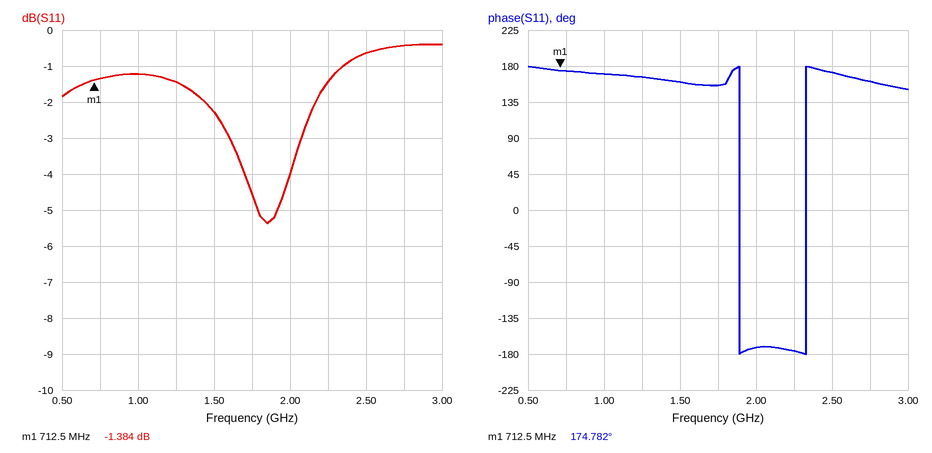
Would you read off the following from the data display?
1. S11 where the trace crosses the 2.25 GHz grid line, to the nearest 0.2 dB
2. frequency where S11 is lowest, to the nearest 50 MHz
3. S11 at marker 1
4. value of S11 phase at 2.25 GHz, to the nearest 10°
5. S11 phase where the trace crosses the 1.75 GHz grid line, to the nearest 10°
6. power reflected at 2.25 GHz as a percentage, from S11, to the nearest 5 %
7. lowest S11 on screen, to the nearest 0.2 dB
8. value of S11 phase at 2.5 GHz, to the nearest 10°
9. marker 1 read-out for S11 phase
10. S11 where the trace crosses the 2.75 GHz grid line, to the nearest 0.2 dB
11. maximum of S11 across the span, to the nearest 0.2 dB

-1.4 dB
1.85 GHz
-1.384 dB
-180°
160°
70 %
-5.4 dB
170°
174.782°
-0.4 dB
-0.4 dB
